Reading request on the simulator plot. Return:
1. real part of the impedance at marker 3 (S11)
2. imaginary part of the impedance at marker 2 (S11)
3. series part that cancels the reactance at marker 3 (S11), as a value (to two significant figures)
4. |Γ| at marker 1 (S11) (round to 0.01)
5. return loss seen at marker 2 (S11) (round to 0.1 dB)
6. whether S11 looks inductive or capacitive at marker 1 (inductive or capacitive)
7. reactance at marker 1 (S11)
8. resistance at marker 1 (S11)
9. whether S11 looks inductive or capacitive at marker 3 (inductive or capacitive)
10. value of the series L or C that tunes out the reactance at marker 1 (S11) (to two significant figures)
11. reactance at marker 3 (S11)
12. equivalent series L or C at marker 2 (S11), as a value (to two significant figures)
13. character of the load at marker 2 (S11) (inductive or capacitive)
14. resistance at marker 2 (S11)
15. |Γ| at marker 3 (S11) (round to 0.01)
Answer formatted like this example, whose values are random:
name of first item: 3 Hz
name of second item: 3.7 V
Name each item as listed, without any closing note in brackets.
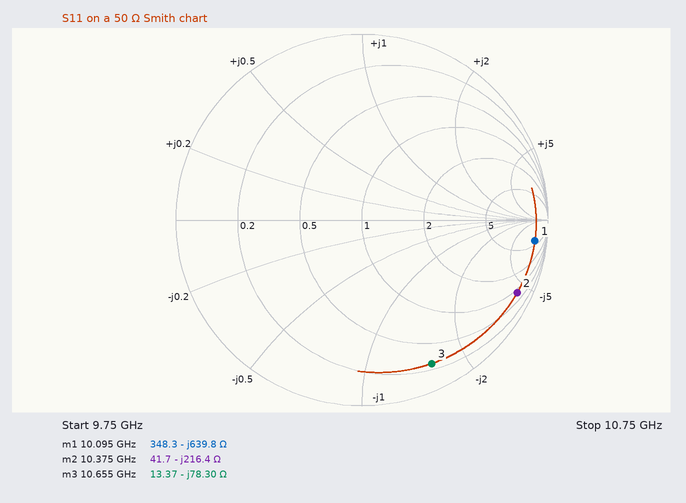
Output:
real part of the impedance at marker 3: 13.37 Ω
imaginary part of the impedance at marker 2: -216.4 Ω
series part that cancels the reactance at marker 3 (S11), as a value: 1.2 nH
|Γ| at marker 1 (S11): 0.94
return loss seen at marker 2 (S11): 0.7 dB
whether S11 looks inductive or capacitive at marker 1: capacitive
reactance at marker 1: -639.8 Ω
resistance at marker 1: 348.3 Ω
whether S11 looks inductive or capacitive at marker 3: capacitive
value of the series L or C that tunes out the reactance at marker 1 (S11): 10 nH
reactance at marker 3: -78.30 Ω
equivalent series L or C at marker 2 (S11), as a value: 71 fF
character of the load at marker 2 (S11): capacitive
resistance at marker 2: 41.7 Ω
|Γ| at marker 3 (S11): 0.86
